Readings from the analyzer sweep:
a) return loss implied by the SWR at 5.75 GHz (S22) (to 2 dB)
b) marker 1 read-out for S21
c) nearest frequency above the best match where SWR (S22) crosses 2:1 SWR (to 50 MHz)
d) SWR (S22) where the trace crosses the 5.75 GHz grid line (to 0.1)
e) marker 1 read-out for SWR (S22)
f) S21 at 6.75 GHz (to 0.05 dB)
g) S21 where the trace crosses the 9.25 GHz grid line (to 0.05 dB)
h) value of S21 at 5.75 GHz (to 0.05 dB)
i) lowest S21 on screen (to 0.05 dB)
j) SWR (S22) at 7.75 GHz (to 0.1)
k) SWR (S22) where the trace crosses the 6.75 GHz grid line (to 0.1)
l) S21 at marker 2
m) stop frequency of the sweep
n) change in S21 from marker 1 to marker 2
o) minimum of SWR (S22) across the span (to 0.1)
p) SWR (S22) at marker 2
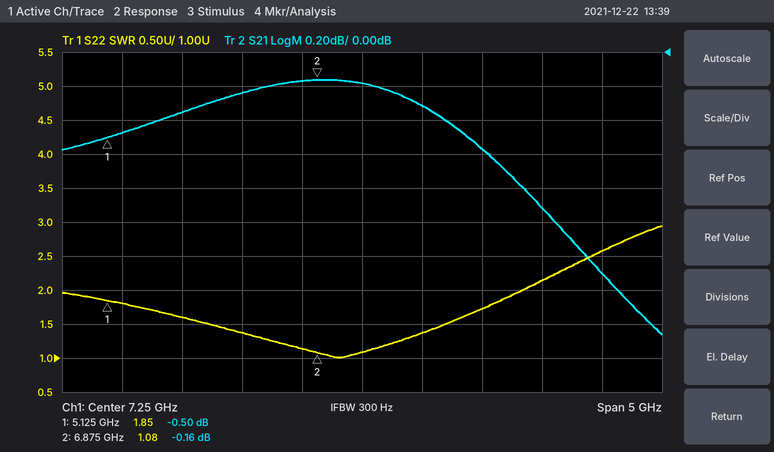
12 dB
-0.50 dB
8.60 GHz
1.6
1.85
-0.15 dB
-1.30 dB
-0.35 dB
-1.65 dB
1.4
1.1
-0.16 dB
9.75 GHz
0.34 dB
1.0
1.08
